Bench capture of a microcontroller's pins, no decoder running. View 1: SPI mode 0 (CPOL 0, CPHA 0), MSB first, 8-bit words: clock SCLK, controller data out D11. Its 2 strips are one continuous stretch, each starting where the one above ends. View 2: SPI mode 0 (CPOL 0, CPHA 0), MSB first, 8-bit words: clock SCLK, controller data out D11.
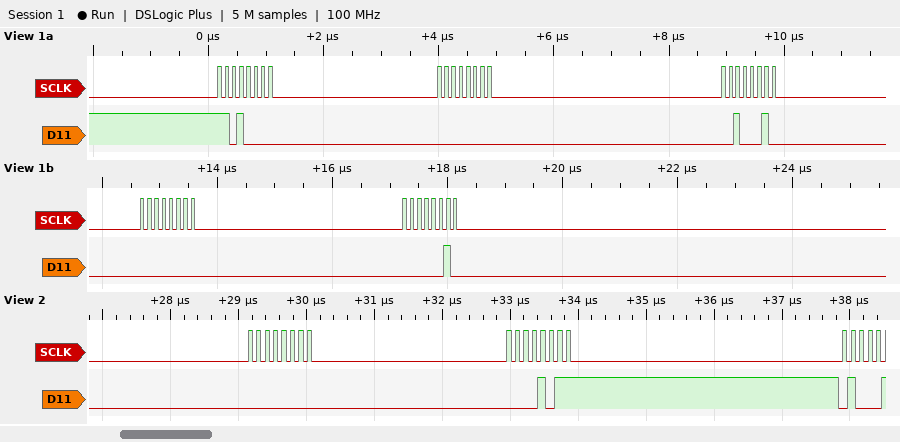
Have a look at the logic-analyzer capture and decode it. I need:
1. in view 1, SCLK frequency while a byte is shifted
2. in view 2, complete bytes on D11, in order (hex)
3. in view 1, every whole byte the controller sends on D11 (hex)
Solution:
8 MHz
00 0B
D0 00 22 00 02
